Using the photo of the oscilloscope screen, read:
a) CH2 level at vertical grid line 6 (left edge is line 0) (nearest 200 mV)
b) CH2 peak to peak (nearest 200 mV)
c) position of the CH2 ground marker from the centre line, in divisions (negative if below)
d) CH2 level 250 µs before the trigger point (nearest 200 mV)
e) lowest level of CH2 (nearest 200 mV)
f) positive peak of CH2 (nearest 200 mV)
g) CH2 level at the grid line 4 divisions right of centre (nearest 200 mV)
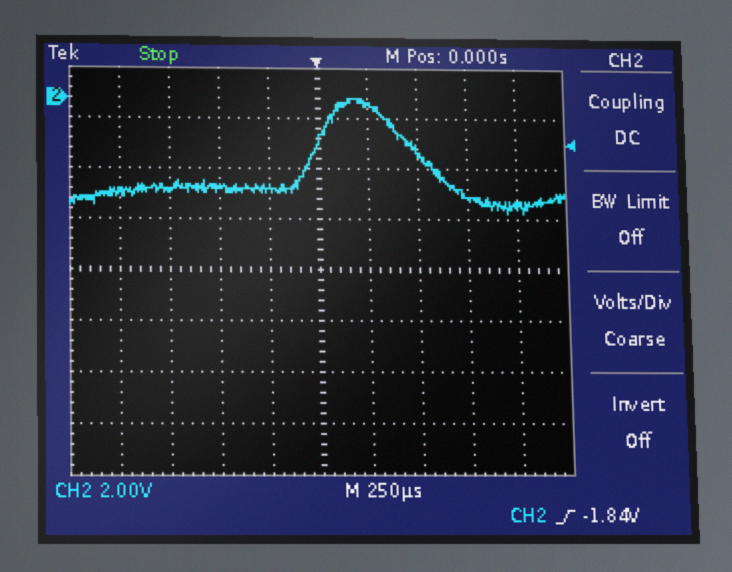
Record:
-200 mV
4.6 V
+3.4 div
-3.6 V
-4.6 V
0.0 V
-4.2 V
